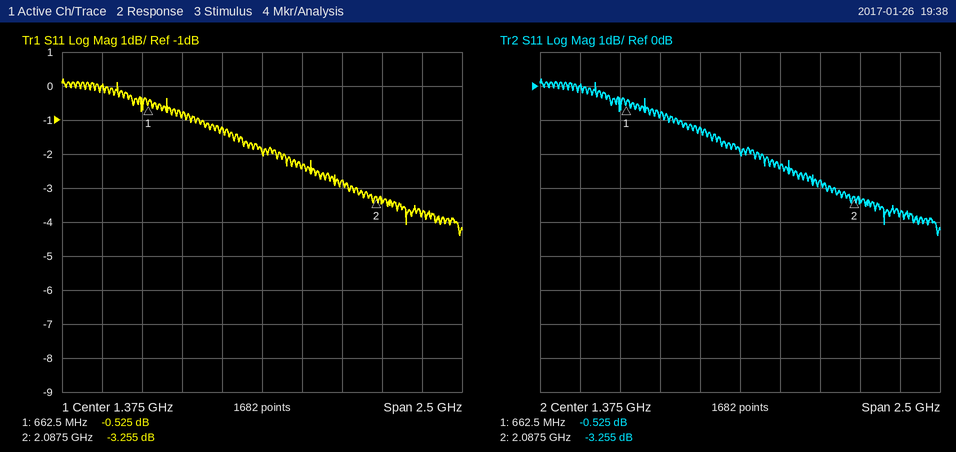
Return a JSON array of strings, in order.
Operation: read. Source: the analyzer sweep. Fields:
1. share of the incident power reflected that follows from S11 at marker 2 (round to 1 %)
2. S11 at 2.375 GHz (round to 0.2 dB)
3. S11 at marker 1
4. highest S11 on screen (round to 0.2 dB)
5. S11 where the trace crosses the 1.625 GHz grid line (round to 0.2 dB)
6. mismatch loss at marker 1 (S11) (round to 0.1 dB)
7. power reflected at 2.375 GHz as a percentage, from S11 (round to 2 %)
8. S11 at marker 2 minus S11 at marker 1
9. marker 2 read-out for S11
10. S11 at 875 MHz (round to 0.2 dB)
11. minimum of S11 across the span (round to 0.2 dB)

["47 %", "-3.8 dB", "-0.525 dB", "0.2 dB", "-2.4 dB", "9.4 dB", "42 %", "-2.730 dB", "-3.255 dB", "-0.8 dB", "-4.4 dB"]
